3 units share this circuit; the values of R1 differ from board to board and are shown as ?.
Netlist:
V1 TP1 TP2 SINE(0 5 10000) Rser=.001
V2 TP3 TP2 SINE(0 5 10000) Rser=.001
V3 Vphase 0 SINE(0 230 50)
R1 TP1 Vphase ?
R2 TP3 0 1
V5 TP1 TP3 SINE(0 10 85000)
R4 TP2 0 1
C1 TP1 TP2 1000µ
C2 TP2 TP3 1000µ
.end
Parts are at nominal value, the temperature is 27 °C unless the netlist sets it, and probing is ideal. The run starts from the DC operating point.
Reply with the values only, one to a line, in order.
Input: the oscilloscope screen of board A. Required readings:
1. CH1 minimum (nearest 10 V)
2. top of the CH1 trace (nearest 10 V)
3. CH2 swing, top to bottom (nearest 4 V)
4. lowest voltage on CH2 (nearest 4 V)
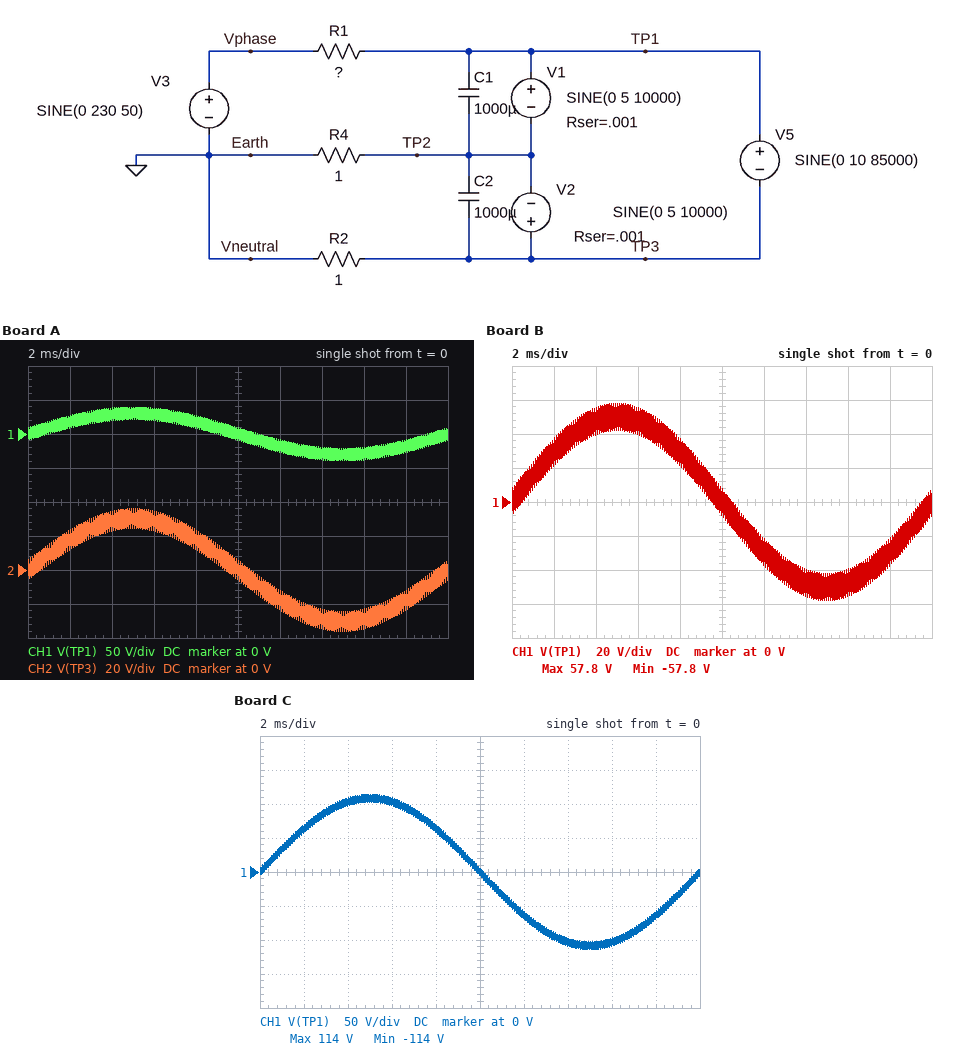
-40 V
40 V
72 V
-36 V
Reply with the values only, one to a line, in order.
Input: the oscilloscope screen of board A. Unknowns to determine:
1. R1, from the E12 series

3.3 Ω
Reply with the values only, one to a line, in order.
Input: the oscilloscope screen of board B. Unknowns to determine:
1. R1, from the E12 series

1.8 Ω
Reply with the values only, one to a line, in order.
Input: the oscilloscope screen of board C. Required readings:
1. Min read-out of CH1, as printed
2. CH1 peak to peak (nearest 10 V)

-114 V
230 V
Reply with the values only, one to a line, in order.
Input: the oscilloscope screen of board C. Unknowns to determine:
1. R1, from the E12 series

0.56 Ω
